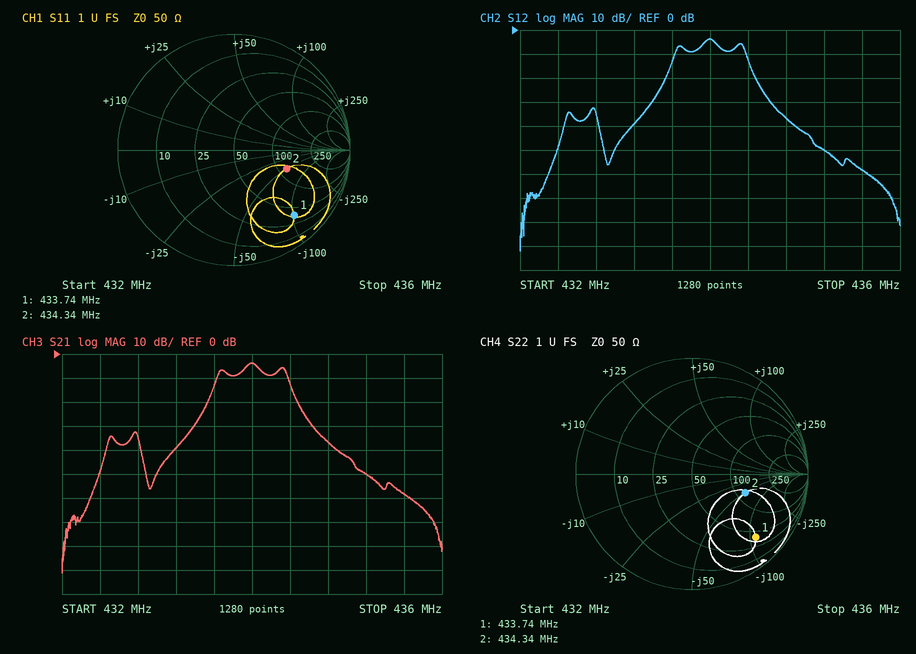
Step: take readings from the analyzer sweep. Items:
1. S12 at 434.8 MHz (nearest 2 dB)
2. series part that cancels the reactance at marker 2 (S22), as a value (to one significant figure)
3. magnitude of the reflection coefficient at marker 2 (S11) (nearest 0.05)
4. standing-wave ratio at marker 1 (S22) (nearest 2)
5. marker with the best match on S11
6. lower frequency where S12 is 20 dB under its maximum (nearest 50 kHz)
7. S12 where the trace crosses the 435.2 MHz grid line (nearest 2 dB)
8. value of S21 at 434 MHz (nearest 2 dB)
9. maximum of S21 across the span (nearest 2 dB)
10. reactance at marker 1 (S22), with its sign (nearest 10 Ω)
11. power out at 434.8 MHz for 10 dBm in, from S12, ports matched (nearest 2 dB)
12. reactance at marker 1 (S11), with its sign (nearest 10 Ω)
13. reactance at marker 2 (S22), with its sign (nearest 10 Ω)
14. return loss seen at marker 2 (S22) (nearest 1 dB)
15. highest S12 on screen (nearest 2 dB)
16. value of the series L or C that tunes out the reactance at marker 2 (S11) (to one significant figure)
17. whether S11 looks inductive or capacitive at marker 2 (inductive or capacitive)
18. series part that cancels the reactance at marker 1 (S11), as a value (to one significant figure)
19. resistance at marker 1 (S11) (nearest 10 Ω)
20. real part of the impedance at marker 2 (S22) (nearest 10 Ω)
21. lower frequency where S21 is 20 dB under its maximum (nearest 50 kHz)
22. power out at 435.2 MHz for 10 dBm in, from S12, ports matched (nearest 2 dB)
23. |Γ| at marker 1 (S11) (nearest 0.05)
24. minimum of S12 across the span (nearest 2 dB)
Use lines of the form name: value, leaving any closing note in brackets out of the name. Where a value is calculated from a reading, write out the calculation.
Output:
S12 at 434.8 MHz: -36 dB
series part that cancels the reactance at marker 2 (S22), as a value: L = 50 Ω/(2π × 434.34 MHz) ≈ 18.3 nH, so 20 nH to one significant figure
magnitude of the reflection coefficient at marker 2 (S11): 0.50
standing-wave ratio at marker 1 (S22): 8
marker with the best match on S11: marker 2
lower frequency where S12 is 20 dB under its maximum: 433.50 MHz
S12 where the trace crosses the 435.2 MHz grid line: -50 dB
value of S21 at 434 MHz: -4 dB
maximum of S21 across the span: -4 dB
reactance at marker 1 (S22), with its sign: -110 Ω
power out at 434.8 MHz for 10 dBm in, from S12, ports matched: 10 dBm + (-36 dB) = -26 dBm
reactance at marker 1 (S11), with its sign: -100 Ω
reactance at marker 2 (S22), with its sign: -50 Ω
return loss seen at marker 2 (S22): 6 dB
highest S12 on screen: -4 dB
value of the series L or C that tunes out the reactance at marker 2 (S11): L = 50 Ω/(2π × 434.34 MHz) ≈ 18.3 nH, so 20 nH to one significant figure
whether S11 looks inductive or capacitive at marker 2: capacitive
series part that cancels the reactance at marker 1 (S11), as a value: L = 100 Ω/(2π × 433.74 MHz) ≈ 36.7 nH, so 40 nH to one significant figure
resistance at marker 1 (S11): 40 Ω
real part of the impedance at marker 2 (S22): 120 Ω
lower frequency where S21 is 20 dB under its maximum: 433.50 MHz
power out at 435.2 MHz for 10 dBm in, from S12, ports matched: 10 dBm + (-50 dB) = -40 dBm
|Γ| at marker 1 (S11): 0.75
minimum of S12 across the span: -92 dB
